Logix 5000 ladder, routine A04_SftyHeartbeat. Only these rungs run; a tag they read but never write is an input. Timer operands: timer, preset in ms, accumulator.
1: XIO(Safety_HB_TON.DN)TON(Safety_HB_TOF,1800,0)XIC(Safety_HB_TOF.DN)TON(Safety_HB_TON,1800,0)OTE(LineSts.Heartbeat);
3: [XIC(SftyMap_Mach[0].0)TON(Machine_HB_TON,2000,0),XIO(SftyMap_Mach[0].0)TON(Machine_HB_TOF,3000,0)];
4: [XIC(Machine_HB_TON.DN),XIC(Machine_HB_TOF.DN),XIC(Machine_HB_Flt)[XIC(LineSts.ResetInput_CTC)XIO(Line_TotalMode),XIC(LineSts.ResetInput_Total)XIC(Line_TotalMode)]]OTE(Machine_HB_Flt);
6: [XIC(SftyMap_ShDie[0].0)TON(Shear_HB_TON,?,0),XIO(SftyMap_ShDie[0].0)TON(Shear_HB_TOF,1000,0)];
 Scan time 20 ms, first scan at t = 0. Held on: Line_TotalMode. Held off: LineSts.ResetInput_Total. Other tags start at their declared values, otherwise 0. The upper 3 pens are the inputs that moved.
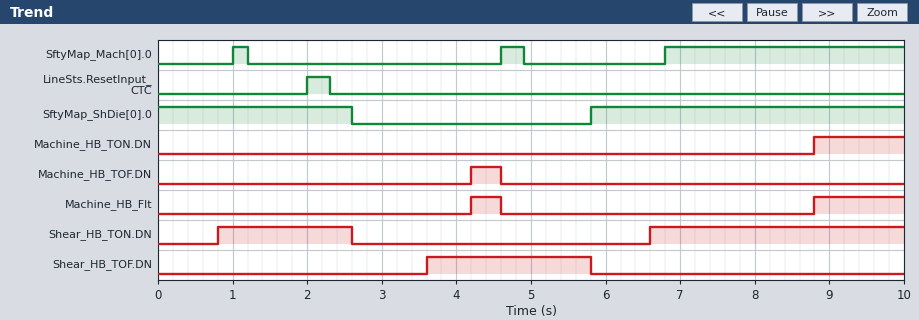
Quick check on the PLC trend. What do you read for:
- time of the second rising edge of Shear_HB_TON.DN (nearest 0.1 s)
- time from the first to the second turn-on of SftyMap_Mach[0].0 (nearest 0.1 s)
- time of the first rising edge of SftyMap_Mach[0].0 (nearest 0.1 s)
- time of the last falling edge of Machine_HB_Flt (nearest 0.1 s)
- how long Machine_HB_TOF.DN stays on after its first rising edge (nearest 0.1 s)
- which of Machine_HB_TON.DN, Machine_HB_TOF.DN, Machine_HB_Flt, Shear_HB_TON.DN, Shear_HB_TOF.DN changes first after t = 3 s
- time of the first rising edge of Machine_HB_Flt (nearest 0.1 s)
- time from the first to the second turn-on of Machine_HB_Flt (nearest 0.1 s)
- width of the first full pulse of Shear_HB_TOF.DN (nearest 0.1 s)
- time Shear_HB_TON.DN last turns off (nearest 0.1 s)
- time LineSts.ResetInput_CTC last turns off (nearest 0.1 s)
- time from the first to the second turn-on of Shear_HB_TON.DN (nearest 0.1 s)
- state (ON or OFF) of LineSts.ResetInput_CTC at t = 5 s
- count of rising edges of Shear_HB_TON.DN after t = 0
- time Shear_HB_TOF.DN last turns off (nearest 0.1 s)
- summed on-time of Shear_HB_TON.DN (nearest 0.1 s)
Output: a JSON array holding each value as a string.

["6.6 s", "3.6 s", "1.0 s", "4.6 s", "0.4 s", "Shear_HB_TOF.DN", "4.2 s", "4.6 s", "2.2 s", "2.6 s", "2.3 s", "5.8 s", "OFF", "2", "5.8 s", "5.2 s"]
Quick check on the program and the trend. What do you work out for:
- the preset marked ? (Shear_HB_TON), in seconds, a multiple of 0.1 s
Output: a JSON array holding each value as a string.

["0.8 s"]
